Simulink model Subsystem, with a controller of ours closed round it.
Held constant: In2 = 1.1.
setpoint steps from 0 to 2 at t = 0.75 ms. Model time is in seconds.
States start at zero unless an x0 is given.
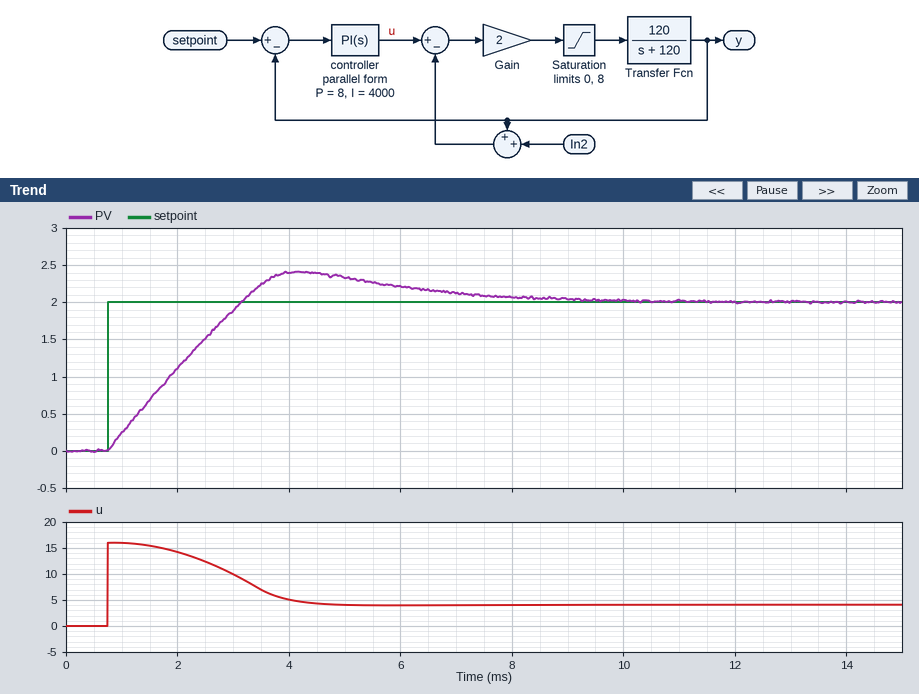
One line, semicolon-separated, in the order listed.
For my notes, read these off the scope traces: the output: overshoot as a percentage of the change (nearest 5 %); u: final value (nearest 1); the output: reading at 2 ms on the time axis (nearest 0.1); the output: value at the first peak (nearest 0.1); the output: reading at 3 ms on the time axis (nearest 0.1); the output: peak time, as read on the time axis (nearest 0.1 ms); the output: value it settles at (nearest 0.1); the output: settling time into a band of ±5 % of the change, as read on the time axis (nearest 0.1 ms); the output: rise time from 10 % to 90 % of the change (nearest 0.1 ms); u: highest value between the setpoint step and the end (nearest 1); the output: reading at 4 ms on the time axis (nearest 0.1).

20 %; 4; 1.1; 2.4; 1.9; 4.2 ms; 2.0; 7.4 ms; 1.9 ms; 16; 2.4
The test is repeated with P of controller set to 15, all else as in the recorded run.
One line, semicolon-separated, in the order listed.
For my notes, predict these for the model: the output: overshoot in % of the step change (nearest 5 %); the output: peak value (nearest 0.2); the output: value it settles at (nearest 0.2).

15 %; 2.2; 2.0
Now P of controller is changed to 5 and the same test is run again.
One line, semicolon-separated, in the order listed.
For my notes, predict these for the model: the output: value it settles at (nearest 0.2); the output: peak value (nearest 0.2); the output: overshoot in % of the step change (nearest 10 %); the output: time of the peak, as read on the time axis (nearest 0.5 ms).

2.0; 2.6; 30 %; 4.5 ms
